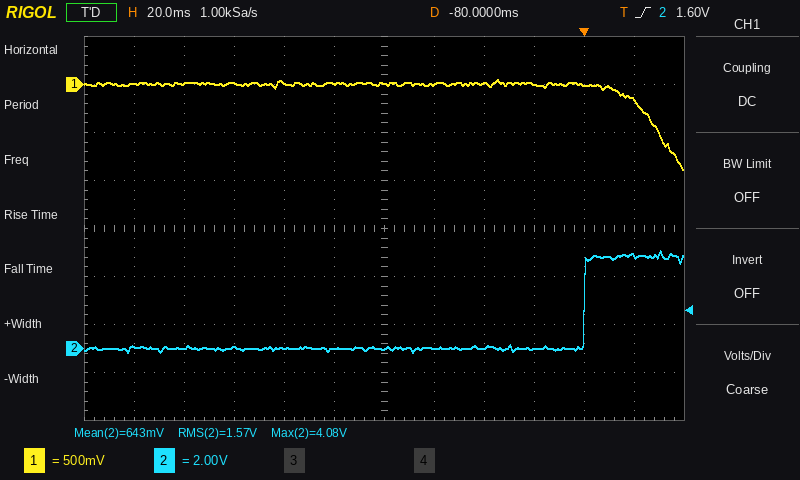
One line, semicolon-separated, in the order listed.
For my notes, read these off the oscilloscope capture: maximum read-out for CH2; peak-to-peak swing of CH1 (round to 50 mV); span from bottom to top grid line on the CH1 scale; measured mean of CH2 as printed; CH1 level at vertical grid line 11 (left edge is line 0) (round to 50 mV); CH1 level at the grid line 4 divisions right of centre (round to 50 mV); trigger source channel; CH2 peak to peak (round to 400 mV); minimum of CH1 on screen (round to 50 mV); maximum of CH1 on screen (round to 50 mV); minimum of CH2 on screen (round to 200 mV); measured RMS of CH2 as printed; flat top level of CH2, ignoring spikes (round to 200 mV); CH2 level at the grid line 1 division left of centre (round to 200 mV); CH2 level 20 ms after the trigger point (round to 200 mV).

4.08 V; 950 mV; 4 V; 643 mV; -150 mV; 0 mV; CH2; 4.4 V; -900 mV; 50 mV; -200 mV; 1.57 V; 3.8 V; 0.0 V; 3.8 V
